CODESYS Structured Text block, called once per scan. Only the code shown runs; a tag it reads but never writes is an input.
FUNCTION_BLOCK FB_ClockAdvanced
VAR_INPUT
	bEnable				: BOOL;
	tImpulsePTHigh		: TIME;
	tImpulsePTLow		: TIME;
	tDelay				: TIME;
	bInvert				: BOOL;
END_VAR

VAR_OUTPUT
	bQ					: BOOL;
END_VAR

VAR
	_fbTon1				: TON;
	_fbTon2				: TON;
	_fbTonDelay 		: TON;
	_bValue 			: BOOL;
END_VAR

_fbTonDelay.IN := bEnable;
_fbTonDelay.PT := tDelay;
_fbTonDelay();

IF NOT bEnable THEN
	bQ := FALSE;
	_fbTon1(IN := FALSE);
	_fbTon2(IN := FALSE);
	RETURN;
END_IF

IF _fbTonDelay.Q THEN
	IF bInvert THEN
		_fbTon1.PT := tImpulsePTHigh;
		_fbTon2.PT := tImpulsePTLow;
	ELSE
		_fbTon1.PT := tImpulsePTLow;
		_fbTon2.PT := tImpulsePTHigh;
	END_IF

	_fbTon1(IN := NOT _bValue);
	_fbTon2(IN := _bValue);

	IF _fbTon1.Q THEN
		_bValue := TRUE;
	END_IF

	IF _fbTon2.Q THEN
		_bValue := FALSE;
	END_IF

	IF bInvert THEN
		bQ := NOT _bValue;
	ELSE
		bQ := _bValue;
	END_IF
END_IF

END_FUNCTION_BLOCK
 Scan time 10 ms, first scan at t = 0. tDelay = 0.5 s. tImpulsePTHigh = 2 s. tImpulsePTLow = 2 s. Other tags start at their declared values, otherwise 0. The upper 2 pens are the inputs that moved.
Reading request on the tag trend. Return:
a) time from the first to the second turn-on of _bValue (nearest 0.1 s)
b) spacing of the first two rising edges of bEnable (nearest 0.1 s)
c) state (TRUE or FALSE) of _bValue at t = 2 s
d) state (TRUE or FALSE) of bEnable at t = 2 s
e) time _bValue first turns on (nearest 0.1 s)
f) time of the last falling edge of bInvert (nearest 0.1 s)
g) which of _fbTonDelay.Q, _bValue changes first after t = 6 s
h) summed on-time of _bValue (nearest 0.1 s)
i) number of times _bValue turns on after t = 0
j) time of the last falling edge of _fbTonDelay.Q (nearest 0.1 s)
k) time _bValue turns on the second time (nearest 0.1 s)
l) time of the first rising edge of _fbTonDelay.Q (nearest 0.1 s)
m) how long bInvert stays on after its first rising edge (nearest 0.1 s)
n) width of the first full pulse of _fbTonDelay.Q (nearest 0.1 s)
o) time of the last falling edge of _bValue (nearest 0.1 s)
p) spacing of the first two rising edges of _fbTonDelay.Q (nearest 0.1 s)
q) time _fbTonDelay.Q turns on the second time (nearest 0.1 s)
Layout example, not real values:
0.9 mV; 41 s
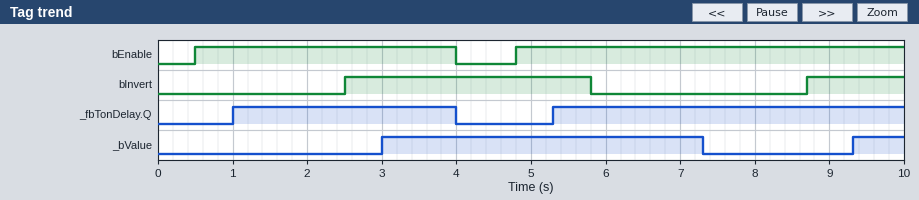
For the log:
6.3 s; 4.3 s; FALSE; TRUE; 3.0 s; 5.8 s; _bValue; 5.0 s; 2; 4.0 s; 9.3 s; 1.0 s; 3.3 s; 3.0 s; 7.3 s; 4.3 s; 5.3 s
